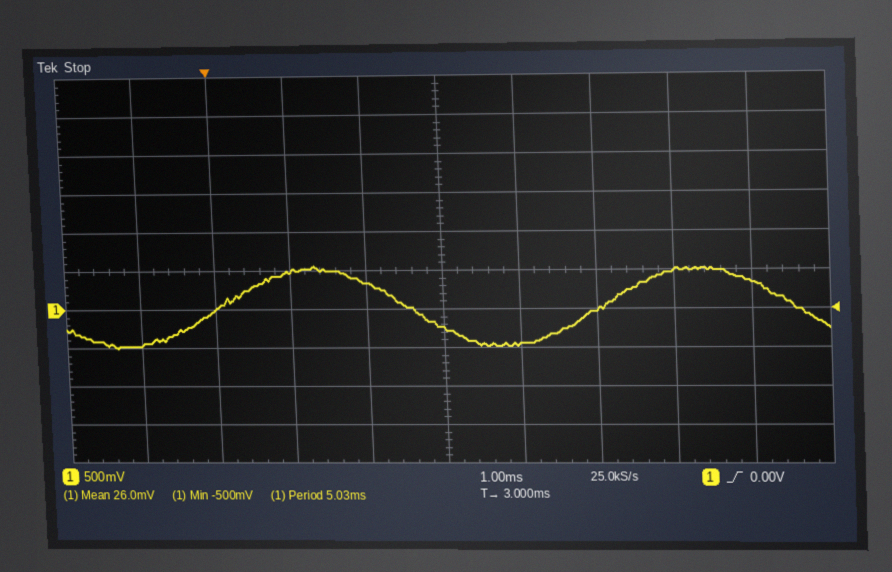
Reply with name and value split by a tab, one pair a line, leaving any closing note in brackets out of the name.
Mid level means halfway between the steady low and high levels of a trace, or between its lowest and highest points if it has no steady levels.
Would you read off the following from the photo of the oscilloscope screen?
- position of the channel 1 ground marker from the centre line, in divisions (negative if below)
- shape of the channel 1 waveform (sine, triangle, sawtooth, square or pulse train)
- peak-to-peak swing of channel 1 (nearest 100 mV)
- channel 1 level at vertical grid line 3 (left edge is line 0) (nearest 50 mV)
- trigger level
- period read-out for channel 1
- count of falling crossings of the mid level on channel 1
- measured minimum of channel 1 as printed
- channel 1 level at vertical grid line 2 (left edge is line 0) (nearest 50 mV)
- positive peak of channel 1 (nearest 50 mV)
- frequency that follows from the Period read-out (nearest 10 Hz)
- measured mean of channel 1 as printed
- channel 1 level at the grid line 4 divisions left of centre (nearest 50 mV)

position of the channel 1 ground marker from the centre line, in divisions	-1.0 div
shape of the channel 1 waveform	sine
peak-to-peak swing of channel 1	1.10 V
channel 1 level at vertical grid line 3 (left edge is line 0)	500 mV
trigger level	0.00 V
period read-out for channel 1	5.03 ms
count of falling crossings of the mid level on channel 1	2
measured minimum of channel 1 as printed	-500 mV
channel 1 level at vertical grid line 2 (left edge is line 0)	0 mV
positive peak of channel 1	550 mV
frequency that follows from the Period read-out	200 Hz
measured mean of channel 1 as printed	26.0 mV
channel 1 level at the grid line 4 divisions left of centre	-450 mV
